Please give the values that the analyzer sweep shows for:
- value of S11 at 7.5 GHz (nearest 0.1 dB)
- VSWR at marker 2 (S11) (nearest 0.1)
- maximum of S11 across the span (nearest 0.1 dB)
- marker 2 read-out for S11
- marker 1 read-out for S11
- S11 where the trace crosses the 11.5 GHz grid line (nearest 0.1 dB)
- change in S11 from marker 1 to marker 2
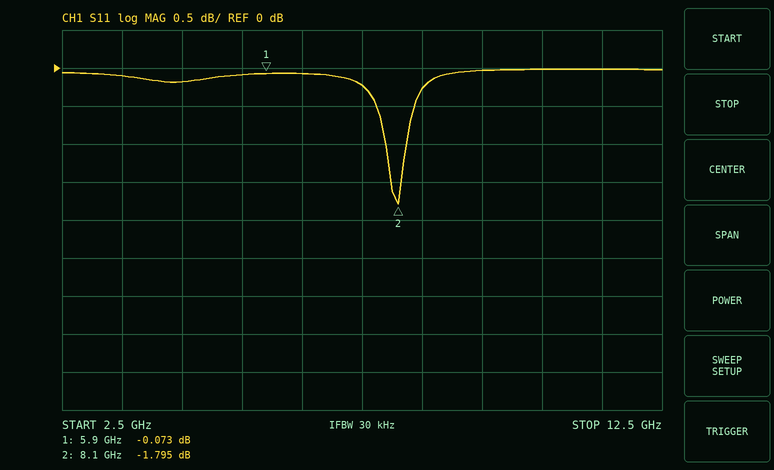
-0.2 dB
9.7
0.0 dB
-1.795 dB
-0.073 dB
0.0 dB
-1.722 dB
